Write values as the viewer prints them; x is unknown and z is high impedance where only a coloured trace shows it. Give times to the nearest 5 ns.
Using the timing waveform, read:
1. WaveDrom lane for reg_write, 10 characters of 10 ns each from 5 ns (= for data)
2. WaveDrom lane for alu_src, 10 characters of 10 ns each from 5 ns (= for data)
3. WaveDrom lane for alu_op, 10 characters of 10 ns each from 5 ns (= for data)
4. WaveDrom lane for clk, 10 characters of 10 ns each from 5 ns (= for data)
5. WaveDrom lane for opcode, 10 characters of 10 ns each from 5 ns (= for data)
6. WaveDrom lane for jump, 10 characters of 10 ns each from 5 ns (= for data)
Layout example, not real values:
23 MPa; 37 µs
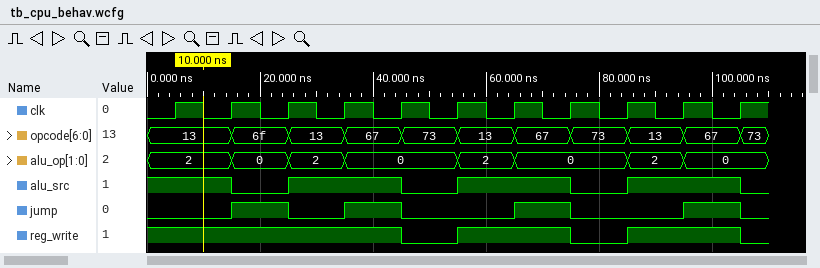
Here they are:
{name: 'reg_write', wave: '1...01.01.'}; {name: 'alu_src', wave: '101.01.01.'}; {name: 'alu_op', wave: '====.==.==', data: '2 0 2 0 2 0 2 0'}; {name: 'clk', wave: 'p.........'}; {name: 'opcode', wave: '==========', data: '13 6f 13 67 73 13 67 73 13 67'}; {name: 'jump', wave: '01010.10.1'}
